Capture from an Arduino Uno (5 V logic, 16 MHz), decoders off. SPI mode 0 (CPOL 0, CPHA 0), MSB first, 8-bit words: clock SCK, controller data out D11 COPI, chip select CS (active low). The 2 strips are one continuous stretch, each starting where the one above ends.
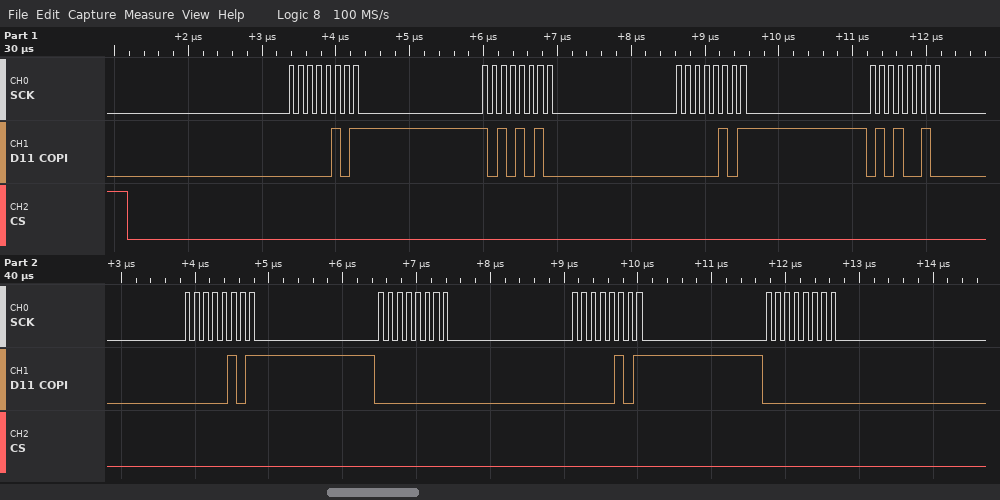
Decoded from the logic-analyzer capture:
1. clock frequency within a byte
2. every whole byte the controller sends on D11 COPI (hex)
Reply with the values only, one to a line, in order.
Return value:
8 MHz
05 AA 05 52 05 00 05 00
